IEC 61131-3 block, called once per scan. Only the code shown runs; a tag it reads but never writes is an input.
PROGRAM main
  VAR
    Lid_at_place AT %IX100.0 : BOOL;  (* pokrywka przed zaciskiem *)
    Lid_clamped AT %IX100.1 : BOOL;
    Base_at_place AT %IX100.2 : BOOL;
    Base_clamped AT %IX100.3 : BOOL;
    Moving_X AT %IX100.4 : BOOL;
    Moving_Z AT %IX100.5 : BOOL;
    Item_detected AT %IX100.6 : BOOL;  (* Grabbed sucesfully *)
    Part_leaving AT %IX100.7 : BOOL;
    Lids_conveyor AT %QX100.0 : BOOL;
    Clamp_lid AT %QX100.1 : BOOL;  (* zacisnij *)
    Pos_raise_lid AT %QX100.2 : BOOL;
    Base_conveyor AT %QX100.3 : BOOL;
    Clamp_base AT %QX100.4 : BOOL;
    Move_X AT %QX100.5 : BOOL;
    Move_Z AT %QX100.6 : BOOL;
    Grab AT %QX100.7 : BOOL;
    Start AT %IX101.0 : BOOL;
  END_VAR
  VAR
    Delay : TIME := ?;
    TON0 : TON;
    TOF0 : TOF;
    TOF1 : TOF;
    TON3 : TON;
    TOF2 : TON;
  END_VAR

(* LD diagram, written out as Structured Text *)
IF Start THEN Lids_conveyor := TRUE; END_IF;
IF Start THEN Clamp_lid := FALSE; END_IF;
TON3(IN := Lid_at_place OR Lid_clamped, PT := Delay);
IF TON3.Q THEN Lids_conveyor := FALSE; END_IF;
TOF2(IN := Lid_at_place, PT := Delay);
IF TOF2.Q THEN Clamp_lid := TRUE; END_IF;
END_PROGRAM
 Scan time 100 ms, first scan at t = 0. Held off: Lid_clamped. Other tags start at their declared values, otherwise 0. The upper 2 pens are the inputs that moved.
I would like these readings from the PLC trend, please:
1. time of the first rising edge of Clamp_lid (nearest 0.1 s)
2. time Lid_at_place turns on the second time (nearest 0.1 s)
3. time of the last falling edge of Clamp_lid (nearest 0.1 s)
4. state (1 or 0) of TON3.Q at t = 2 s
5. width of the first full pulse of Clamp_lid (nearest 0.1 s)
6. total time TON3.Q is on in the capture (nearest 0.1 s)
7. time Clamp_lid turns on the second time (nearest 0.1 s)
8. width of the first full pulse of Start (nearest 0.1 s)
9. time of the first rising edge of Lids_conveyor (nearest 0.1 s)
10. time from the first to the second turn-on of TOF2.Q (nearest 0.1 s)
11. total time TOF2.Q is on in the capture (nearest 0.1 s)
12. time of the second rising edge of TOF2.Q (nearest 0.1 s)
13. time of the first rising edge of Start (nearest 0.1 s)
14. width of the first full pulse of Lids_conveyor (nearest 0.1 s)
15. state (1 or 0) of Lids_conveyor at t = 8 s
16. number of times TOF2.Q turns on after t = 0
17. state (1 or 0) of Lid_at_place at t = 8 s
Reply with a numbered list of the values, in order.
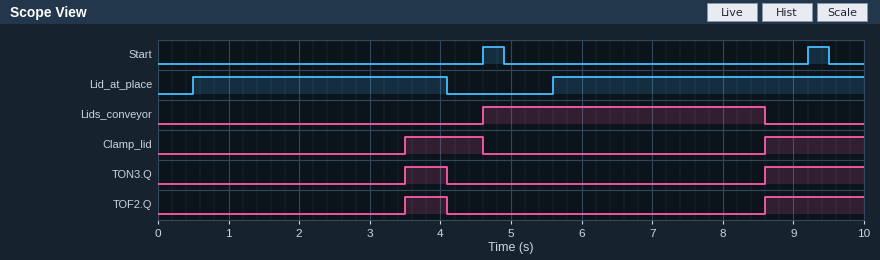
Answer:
1. 3.5 s
2. 5.6 s
3. 4.6 s
4. 0
5. 1.1 s
6. 2.0 s
7. 8.6 s
8. 0.3 s
9. 4.6 s
10. 5.1 s
11. 2.0 s
12. 8.6 s
13. 4.6 s
14. 4.0 s
15. 1
16. 2
17. 1
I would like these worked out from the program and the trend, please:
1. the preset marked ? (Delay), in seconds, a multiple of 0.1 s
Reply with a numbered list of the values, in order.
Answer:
1. 3.0 s
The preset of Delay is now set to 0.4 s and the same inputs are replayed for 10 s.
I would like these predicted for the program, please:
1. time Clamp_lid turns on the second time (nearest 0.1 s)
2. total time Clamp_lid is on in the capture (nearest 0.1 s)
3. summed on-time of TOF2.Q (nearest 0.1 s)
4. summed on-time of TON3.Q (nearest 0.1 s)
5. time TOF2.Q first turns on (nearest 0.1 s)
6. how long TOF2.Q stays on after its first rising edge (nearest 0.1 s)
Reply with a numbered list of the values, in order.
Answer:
1. 6.0 s
2. 7.7 s
3. 7.2 s
4. 7.2 s
5. 0.9 s
6. 3.2 s
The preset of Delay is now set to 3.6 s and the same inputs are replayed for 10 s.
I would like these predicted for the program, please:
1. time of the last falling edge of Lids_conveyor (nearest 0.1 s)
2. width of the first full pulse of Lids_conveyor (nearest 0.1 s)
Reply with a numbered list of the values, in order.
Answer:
1. 9.2 s
2. 4.6 s
